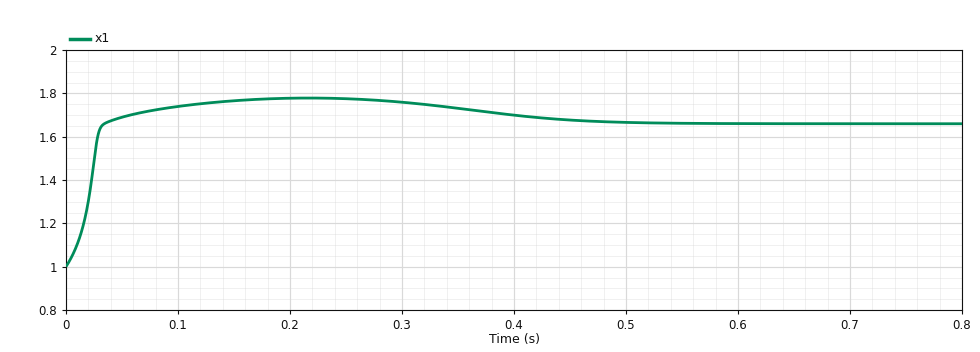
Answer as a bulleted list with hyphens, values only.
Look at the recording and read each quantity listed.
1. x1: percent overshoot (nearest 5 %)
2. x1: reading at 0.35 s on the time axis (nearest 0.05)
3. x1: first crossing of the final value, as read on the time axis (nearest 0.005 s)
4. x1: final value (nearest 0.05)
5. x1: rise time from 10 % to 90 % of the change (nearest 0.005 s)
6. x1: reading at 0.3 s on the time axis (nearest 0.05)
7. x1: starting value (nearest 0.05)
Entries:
- 20 %
- 1.75
- 0.035 s
- 1.65
- 0.020 s
- 1.75
- 1.00
